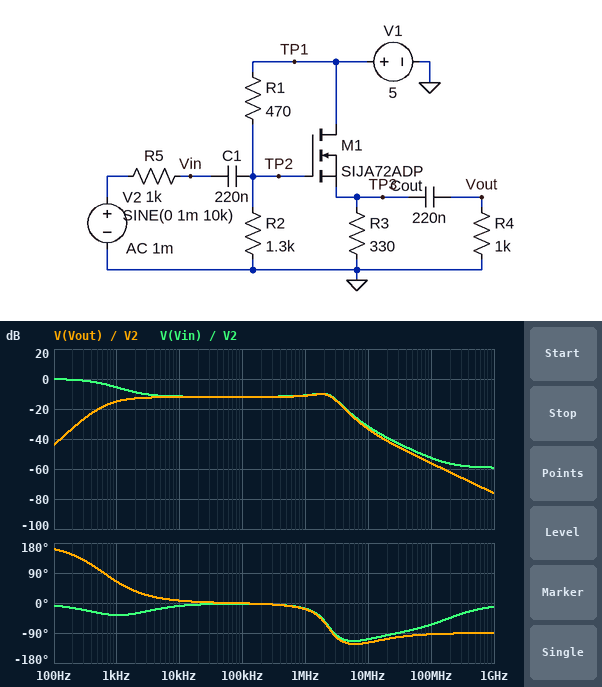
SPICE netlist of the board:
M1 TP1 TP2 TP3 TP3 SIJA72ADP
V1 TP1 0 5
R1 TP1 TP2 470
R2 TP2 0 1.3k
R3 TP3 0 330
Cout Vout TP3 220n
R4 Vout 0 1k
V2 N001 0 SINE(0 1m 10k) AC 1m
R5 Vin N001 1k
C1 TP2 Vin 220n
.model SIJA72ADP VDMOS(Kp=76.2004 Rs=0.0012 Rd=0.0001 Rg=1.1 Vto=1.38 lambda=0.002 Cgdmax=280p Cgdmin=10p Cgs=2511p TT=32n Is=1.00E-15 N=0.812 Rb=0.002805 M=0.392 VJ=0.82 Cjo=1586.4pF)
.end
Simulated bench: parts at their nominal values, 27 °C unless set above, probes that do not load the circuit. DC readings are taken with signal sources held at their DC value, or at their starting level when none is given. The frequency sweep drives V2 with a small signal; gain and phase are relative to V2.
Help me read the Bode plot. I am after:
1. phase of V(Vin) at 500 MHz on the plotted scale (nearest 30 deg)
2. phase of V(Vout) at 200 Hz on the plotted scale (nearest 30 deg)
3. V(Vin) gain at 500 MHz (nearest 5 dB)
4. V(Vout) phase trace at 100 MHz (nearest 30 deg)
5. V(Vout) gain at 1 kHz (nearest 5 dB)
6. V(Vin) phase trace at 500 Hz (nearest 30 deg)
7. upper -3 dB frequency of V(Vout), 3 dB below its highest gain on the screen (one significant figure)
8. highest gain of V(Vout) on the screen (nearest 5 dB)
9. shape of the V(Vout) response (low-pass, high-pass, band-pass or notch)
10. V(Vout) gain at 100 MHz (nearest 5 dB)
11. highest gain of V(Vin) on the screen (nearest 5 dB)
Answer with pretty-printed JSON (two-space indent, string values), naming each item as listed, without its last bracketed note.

{
  "phase of V(Vin) at 500 MHz on the plotted scale": "-30 deg",
  "phase of V(Vout) at 200 Hz on the plotted scale": "150 deg",
  "V(Vin) gain at 500 MHz": "-60 dB",
  "V(Vout) phase trace at 100 MHz": "-90 deg",
  "V(Vout) gain at 1 kHz": "-15 dB",
  "V(Vin) phase trace at 500 Hz": "-30 deg",
  "upper -3 dB frequency of V(Vout), 3 dB below its highest gain on the screen": "3 MHz",
  "highest gain of V(Vout) on the screen": "-10 dB",
  "shape of the V(Vout) response": "band-pass",
  "V(Vout) gain at 100 MHz": "-55 dB",
  "highest gain of V(Vin) on the screen": "0 dB"
}
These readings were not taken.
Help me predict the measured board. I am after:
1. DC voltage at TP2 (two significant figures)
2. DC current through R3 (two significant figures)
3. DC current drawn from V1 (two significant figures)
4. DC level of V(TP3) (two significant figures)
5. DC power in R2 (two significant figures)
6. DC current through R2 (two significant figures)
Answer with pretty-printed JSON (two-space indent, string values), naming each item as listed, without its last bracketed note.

{
  "DC voltage at TP2": "3.7 V",
  "DC current through R3": "7.5 mA",
  "DC current drawn from V1": "10 mA",
  "DC level of V(TP3)": "2.5 V",
  "DC power in R2": "10 mW",
  "DC current through R2": "2.8 mA"
}
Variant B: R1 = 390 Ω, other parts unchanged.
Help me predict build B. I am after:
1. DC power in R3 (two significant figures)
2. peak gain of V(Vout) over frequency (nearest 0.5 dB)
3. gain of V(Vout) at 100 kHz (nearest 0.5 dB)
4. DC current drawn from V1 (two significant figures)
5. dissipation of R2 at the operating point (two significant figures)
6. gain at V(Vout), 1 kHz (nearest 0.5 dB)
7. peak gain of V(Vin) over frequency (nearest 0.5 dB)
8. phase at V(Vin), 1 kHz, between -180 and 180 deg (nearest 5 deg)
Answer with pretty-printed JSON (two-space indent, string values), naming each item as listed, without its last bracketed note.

{
  "DC power in R3": "21 mW",
  "peak gain of V(Vout) over frequency": "-11.0 dB",
  "gain of V(Vout) at 100 kHz": "-13.0 dB",
  "DC current drawn from V1": "11 mA",
  "dissipation of R2 at the operating point": "11 mW",
  "gain at V(Vout), 1 kHz": "-16.0 dB",
  "peak gain of V(Vin) over frequency": "0 dB",
  "phase at V(Vin), 1 kHz, between -180 and 180 deg": "-40 deg"
}
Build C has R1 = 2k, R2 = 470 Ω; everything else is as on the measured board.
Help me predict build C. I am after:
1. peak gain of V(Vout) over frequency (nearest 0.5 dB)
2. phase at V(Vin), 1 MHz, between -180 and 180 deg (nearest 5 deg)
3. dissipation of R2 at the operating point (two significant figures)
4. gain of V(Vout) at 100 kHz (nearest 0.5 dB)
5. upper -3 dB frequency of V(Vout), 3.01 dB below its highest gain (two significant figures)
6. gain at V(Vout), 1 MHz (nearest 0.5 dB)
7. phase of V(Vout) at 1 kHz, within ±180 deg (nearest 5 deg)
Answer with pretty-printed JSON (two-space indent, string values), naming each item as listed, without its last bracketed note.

{
  "peak gain of V(Vout) over frequency": "-19.0 dB",
  "phase at V(Vin), 1 MHz, between -180 and 180 deg": "-35 deg",
  "dissipation of R2 at the operating point": "1.9 mW",
  "gain of V(Vout) at 100 kHz": "-21.5 dB",
  "upper -3 dB frequency of V(Vout), 3.01 dB below its highest gain": "1.9 MHz",
  "gain at V(Vout), 1 MHz": "-19.5 dB",
  "phase of V(Vout) at 1 kHz, within ±180 deg": "60 deg"
}
